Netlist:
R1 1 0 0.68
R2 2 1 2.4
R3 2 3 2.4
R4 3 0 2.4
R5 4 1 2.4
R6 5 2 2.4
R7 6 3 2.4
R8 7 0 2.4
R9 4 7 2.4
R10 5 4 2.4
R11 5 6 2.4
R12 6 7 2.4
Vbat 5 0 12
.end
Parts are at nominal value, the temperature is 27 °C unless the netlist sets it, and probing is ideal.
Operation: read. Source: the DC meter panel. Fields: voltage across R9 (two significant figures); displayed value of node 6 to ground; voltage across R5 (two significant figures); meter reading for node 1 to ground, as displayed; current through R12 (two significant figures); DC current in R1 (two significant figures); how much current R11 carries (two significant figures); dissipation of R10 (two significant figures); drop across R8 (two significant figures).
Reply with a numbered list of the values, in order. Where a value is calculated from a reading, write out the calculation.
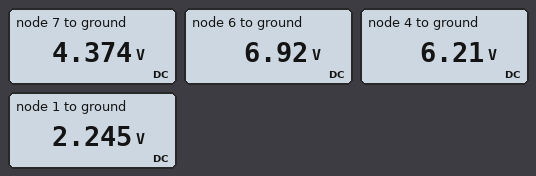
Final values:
1. 6.21 V - 4.374 V = 1.8 V
2. 6.92 V
3. 6.21 V - 2.245 V = 4.0 V
4. 2.245 V
5. (6.92 V - 4.374 V) / 2.4 Ω = 1.1 A
6. (2.245 V) / 680 mΩ = 3.3 A
7. (12 V - 6.92 V) / 2.4 Ω = 2.1 A
8. (12 V - 6.21 V)^2 / 2.4 Ω = 14 W
9. 4.374 V = 4.4 V
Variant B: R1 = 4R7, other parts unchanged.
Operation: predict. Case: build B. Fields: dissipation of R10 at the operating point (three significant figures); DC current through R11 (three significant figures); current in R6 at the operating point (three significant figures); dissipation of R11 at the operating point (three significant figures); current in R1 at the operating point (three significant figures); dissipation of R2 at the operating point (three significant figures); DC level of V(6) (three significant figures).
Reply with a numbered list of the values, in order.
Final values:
1. 7.61 W
2. 1.94 A
3. 1.78 A
4. 9.01 W
5. 1.31 A
6. 1.03 W
7. 7.35 V
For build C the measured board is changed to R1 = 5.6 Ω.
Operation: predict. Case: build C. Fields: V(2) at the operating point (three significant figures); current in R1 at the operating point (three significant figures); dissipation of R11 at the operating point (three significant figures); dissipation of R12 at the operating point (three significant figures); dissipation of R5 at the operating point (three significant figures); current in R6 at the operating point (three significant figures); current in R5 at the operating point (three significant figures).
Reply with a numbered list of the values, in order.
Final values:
1. 7.85 V
2. 1.15 A
3. 8.88 W
4. 2.22 W
5. 799 mW
6. 1.73 A
7. 577 mA
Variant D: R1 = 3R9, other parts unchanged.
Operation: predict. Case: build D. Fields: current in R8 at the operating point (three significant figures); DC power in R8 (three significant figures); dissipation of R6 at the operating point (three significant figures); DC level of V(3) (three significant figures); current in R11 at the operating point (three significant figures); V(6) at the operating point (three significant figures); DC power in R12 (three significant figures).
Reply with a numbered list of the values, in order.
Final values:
1. 2.07 A
2. 10.3 W
3. 8.10 W
4. 4.97 V
5. 1.95 A
6. 7.31 V
7. 2.29 W
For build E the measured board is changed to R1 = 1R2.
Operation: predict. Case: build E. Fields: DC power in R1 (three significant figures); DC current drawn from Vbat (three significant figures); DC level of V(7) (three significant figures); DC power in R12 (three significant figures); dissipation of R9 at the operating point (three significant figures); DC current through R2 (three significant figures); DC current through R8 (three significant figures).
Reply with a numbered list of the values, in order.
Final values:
1. 9.13 W
2. 6.55 A
3. 4.55 V
4. 2.57 W
5. 1.78 W
6. 1.38 A
7. 1.90 A
